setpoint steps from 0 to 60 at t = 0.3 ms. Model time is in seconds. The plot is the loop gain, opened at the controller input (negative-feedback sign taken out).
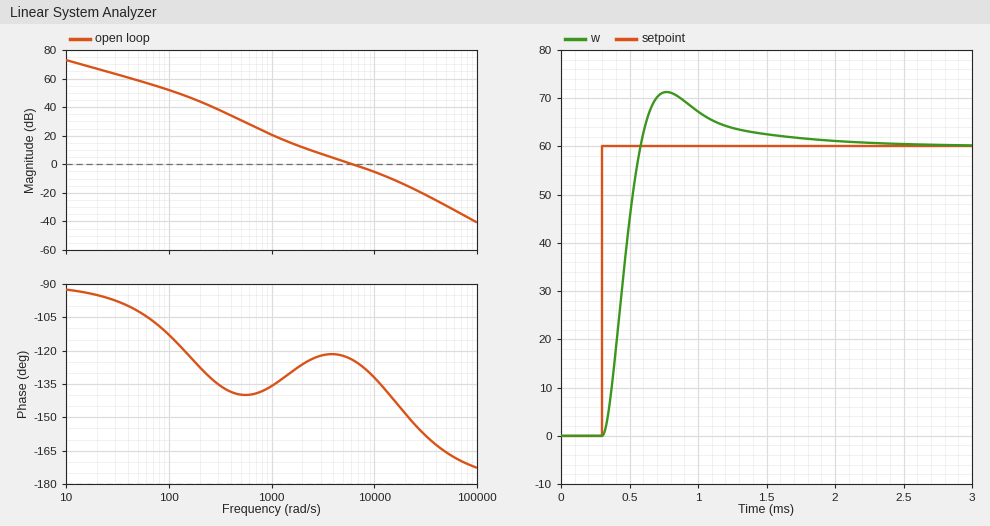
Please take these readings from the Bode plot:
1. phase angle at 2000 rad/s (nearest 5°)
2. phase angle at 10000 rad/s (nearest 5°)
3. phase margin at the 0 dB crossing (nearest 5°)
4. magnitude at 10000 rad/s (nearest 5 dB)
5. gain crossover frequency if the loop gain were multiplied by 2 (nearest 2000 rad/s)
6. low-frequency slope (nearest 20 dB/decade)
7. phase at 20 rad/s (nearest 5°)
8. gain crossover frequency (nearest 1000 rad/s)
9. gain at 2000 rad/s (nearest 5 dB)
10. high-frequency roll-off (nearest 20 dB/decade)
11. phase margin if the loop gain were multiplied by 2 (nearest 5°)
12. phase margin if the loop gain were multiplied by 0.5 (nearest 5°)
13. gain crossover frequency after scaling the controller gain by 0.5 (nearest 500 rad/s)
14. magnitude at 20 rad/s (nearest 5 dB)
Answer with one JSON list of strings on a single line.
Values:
["-125°", "-130°", "55°", "-5 dB", "10000 rad/s", "-20 dB/decade", "-95°", "6000 rad/s", "10 dB", "-40 dB/decade", "45°", "60°", "3500 rad/s", "65 dB"]
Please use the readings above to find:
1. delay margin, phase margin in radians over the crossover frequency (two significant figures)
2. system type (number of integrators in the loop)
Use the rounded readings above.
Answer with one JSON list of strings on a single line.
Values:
["0.00016 s", "1"]
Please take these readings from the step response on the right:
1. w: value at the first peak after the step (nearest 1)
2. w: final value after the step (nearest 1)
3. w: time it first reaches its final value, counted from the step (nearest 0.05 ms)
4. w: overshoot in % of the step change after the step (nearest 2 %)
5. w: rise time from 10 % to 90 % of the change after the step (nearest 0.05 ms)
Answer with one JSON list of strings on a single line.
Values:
["71", "60", "0.30 ms", "18 %", "0.20 ms"]
